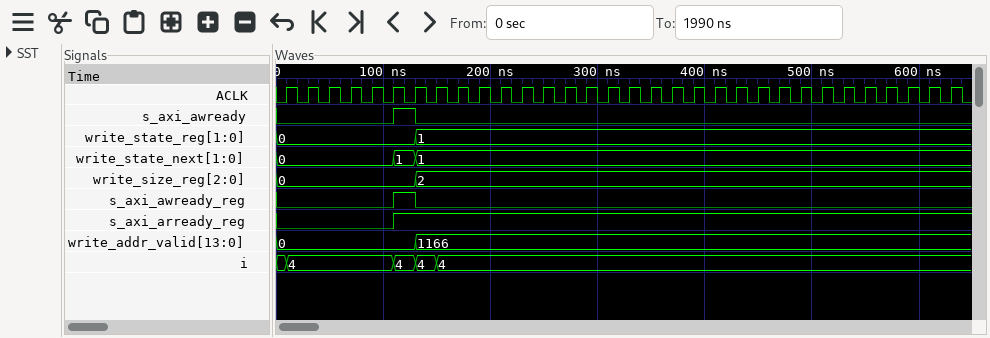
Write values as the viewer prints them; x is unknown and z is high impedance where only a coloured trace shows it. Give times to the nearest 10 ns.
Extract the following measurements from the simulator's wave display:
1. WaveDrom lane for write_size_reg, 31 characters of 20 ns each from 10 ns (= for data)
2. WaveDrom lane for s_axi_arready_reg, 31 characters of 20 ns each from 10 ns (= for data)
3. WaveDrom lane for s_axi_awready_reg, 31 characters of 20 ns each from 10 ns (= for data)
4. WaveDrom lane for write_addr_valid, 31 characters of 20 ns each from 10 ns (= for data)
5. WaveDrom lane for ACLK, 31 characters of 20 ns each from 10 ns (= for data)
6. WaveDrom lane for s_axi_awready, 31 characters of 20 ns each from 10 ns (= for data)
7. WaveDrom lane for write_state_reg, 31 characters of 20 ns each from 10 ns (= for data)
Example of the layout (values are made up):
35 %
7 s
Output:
{name: 'write_size_reg', wave: '=.....=........................', data: '0 2'}
{name: 's_axi_arready_reg', wave: '0....1.........................'}
{name: 's_axi_awready_reg', wave: '0....10........................'}
{name: 'write_addr_valid', wave: '=.....=........................', data: '0 1166'}
{name: 'ACLK', wave: 'p..............................'}
{name: 's_axi_awready', wave: '0....10........................'}
{name: 'write_state_reg', wave: '=.....=........................', data: '0 1'}
